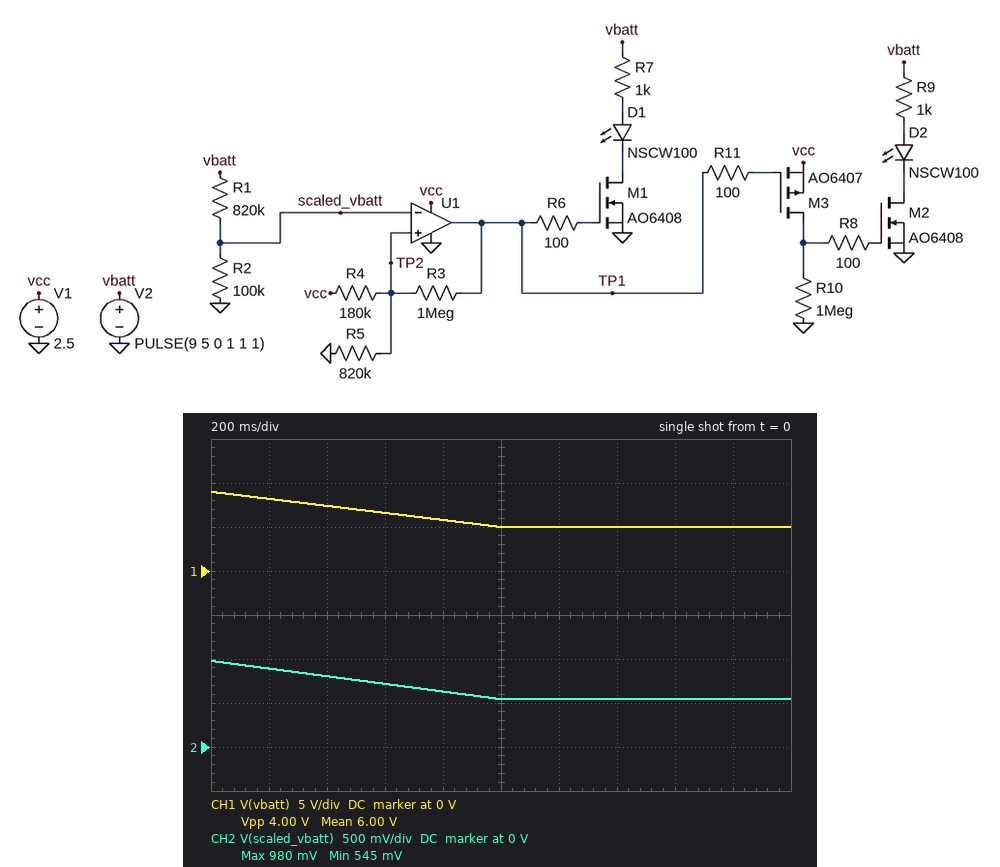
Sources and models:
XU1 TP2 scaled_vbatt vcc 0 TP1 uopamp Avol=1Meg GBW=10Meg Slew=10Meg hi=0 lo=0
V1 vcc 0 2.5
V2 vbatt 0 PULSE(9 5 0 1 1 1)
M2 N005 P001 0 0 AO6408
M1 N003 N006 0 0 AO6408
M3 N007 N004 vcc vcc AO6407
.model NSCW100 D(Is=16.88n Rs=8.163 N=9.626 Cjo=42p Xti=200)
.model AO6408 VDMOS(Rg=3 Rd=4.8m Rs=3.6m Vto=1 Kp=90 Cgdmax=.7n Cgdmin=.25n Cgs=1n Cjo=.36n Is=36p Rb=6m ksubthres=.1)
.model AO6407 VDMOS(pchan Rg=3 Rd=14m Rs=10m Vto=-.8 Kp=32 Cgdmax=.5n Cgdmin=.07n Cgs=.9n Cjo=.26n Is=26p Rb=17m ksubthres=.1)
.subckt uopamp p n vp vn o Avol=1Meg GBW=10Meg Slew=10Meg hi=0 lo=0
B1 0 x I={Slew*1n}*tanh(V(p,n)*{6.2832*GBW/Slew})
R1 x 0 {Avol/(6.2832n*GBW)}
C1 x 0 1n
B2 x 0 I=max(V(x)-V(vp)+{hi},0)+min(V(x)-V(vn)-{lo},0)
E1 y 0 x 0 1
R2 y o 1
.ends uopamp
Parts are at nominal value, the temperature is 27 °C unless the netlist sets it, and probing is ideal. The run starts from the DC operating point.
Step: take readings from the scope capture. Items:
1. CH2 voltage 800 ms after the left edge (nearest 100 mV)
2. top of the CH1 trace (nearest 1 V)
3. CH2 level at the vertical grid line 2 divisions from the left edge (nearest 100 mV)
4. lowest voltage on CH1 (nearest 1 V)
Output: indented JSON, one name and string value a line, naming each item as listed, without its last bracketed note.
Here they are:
{
  "CH2 voltage 800 ms after the left edge": "600 mV",
  "top of the CH1 trace": "9 V",
  "CH2 level at the vertical grid line 2 divisions from the left edge": "800 mV",
  "lowest voltage on CH1": "5 V"
}
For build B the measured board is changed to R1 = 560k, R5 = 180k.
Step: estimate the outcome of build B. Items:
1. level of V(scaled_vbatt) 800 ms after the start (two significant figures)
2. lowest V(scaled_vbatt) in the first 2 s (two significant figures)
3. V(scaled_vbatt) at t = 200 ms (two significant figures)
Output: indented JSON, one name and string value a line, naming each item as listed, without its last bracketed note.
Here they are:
{
  "level of V(scaled_vbatt) 800 ms after the start": "880 mV",
  "lowest V(scaled_vbatt) in the first 2 s": "760 mV",
  "V(scaled_vbatt) at t = 200 ms": "1.2 V"
}
